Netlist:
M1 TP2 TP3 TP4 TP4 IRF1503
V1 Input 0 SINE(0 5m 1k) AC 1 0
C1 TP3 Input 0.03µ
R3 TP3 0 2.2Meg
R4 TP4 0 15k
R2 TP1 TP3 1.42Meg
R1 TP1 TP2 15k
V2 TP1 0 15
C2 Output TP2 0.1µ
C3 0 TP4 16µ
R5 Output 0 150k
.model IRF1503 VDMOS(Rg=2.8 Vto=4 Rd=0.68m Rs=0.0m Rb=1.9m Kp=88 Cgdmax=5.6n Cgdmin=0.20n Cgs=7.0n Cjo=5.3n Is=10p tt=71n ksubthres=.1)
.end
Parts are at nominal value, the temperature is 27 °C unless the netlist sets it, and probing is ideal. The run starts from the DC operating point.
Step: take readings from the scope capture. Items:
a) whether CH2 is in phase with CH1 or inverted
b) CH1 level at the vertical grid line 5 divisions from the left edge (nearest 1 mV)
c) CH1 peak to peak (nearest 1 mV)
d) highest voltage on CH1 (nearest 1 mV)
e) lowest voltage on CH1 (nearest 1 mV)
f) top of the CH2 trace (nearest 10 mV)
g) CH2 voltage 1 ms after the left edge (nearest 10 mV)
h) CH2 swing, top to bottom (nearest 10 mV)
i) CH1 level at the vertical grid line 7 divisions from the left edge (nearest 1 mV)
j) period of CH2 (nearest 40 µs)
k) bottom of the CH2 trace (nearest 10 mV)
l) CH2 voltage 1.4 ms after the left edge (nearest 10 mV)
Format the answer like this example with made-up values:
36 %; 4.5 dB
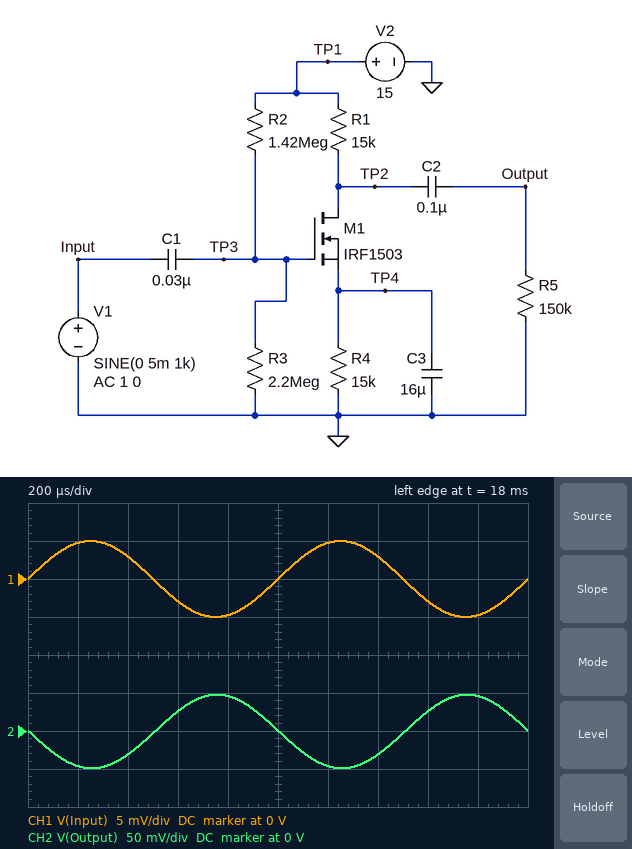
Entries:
inverted; 0 V; 10 mV; 5 mV; -5 mV; 50 mV; 0 V; 100 mV; 3 mV; 1.00 ms; -50 mV; -30 mV
